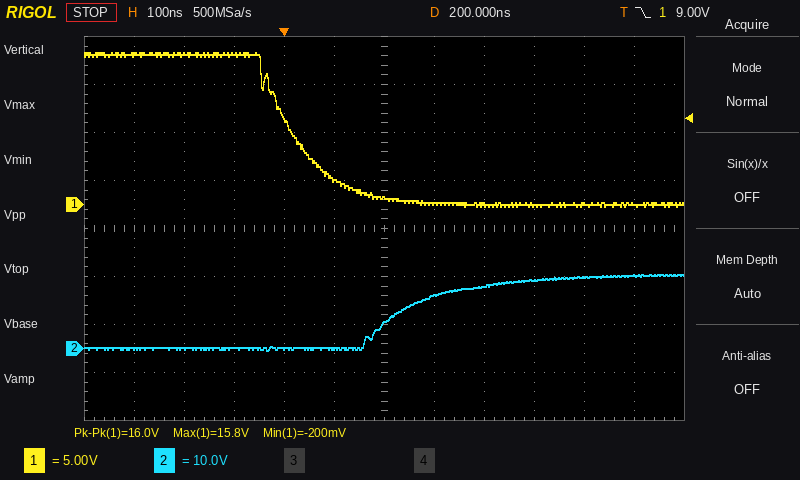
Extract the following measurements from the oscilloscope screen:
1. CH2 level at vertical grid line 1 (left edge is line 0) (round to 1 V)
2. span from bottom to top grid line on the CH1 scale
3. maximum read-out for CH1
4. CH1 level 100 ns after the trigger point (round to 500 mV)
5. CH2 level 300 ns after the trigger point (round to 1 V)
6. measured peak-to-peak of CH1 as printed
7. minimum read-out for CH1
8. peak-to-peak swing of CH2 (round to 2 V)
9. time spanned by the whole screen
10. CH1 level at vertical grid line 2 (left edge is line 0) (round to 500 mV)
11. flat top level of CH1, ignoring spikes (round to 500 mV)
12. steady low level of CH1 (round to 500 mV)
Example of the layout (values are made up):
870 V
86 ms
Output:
0 V
40 V
15.8 V
2.5 V
11 V
16.0 V
-200 mV
16 V
1.2 µs
15.5 V
15.5 V
0.0 V
